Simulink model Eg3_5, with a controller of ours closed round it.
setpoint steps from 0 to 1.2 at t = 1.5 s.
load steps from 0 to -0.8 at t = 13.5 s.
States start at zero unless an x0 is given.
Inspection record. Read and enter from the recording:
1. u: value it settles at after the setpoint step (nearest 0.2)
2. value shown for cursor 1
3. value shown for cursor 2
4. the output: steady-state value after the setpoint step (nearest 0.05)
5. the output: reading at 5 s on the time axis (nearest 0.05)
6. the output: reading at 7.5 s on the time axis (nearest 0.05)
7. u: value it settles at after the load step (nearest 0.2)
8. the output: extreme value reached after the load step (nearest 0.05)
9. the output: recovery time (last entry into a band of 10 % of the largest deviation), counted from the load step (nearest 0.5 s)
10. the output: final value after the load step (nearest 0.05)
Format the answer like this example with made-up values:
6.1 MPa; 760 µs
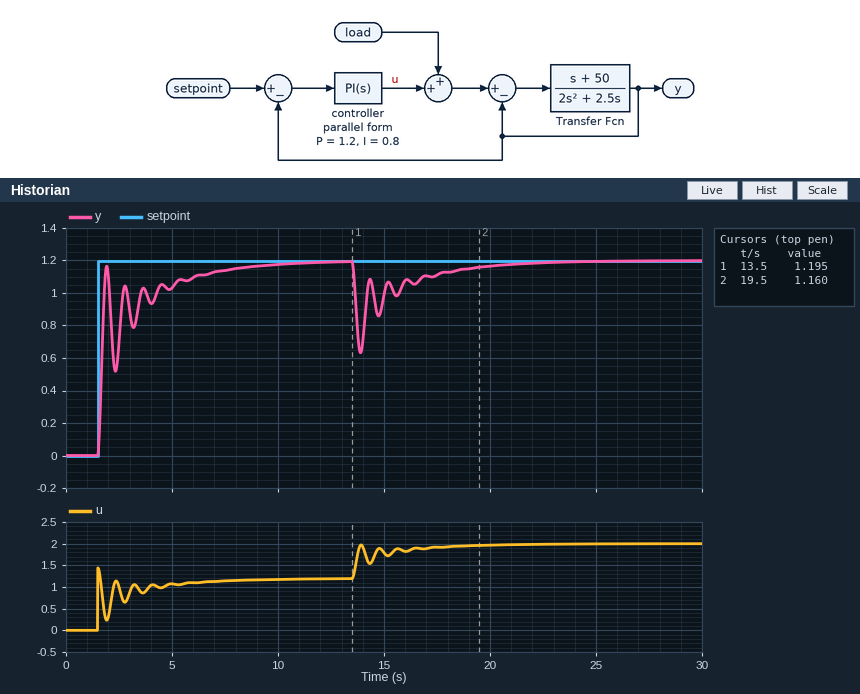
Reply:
1.2; 1.195; 1.160; 1.20; 1.05; 1.15; 2.0; 0.65; 5.0 s; 1.20
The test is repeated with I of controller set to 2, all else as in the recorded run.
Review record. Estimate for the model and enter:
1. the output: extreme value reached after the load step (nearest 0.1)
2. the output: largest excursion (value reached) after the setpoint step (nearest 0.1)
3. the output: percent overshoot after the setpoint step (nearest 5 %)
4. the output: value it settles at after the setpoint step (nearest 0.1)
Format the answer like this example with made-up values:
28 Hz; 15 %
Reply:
0.7; 1.3; 10 %; 1.2
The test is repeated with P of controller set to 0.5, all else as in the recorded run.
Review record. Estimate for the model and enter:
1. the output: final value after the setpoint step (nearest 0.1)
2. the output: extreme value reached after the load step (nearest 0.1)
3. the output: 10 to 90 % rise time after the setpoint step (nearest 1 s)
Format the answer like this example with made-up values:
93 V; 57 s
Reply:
1.2; 0.4; 3 s
